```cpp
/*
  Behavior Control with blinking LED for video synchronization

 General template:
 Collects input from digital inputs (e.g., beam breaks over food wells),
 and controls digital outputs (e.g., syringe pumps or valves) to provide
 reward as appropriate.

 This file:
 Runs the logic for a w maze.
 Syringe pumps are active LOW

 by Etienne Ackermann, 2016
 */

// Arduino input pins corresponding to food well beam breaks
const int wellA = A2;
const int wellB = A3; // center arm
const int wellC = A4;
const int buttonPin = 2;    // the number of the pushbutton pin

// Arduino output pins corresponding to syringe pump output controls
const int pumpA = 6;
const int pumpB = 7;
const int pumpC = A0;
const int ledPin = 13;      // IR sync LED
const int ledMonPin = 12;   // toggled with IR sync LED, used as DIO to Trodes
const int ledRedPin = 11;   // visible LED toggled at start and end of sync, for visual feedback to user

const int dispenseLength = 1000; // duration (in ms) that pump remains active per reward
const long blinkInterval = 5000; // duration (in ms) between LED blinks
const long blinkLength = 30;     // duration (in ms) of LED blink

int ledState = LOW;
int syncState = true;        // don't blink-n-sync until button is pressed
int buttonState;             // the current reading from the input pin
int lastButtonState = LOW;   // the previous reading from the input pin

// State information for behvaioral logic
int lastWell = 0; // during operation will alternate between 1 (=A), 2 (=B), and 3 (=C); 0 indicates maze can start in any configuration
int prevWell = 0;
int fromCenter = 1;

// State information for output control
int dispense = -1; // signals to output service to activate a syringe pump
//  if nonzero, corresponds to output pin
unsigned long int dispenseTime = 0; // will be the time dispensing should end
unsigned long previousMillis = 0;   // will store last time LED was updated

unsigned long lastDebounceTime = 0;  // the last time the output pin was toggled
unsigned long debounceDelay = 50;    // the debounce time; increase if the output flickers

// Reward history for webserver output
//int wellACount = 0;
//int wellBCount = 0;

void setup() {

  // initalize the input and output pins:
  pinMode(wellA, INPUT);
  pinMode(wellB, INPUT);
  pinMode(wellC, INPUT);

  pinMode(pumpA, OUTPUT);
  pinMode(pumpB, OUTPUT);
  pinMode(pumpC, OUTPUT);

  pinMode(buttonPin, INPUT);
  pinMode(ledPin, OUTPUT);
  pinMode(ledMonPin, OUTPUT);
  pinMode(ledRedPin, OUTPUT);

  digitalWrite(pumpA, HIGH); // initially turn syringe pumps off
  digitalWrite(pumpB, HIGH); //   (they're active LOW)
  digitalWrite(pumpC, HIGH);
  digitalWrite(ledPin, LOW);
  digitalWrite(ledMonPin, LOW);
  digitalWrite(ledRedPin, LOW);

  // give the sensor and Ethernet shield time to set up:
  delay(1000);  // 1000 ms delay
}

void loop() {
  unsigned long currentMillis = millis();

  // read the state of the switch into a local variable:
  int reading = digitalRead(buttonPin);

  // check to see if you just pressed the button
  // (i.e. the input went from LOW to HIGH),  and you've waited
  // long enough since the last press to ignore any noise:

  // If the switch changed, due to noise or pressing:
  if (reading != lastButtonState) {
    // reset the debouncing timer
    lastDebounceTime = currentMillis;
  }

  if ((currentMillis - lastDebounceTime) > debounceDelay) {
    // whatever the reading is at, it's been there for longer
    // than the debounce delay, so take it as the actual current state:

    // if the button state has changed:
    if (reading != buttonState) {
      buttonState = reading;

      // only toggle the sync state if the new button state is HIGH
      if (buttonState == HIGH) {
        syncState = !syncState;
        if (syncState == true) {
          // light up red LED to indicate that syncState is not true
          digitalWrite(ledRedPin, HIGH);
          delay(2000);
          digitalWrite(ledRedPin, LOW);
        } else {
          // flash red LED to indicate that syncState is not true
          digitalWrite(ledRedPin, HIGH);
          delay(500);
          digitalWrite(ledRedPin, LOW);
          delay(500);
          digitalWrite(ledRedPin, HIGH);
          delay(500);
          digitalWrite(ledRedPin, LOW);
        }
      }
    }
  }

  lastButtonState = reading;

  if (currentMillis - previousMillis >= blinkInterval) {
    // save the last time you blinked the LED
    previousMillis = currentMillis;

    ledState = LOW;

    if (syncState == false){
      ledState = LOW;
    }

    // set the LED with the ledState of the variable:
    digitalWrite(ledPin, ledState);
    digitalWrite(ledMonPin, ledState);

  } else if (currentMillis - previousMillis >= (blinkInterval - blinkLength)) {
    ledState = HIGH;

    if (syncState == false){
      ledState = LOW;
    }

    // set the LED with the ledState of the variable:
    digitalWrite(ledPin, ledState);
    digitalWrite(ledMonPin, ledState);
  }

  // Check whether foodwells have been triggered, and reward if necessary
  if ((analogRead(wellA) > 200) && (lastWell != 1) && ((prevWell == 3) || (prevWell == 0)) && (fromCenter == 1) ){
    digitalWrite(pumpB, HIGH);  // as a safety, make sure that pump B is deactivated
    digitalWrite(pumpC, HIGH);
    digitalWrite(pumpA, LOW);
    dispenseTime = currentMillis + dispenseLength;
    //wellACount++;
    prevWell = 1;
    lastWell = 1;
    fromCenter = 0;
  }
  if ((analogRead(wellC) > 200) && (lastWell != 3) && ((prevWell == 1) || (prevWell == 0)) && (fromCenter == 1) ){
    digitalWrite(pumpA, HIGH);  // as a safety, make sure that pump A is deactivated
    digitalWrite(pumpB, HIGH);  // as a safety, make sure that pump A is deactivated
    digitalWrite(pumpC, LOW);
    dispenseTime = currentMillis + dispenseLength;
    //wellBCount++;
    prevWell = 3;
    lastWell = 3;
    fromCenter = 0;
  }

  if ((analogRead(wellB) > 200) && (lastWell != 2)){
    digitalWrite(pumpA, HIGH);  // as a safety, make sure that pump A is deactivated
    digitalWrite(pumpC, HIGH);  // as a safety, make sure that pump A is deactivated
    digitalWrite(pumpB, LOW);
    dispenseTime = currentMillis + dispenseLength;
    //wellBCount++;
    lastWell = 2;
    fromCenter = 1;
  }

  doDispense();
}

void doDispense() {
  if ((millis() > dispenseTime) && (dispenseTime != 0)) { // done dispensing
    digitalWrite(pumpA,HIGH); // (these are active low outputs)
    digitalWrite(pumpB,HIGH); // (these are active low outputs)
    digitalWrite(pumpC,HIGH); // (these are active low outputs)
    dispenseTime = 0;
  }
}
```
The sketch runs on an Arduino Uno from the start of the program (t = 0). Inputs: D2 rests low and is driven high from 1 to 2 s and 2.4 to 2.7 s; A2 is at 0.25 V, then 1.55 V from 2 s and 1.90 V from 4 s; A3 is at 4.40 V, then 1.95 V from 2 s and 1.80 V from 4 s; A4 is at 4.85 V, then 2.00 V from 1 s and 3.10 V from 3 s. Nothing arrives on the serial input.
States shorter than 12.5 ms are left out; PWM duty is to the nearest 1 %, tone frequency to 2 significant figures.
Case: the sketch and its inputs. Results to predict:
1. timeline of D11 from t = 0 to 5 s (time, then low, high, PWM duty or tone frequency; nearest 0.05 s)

0 s low; 1.05 s high; 1.55 s low; 2.05 s high; 2.55 s low
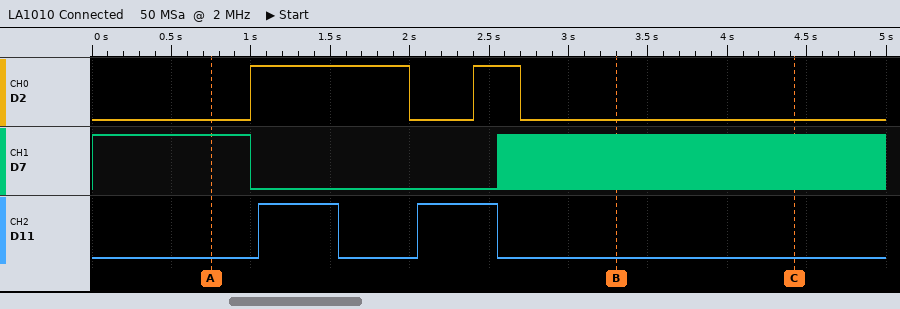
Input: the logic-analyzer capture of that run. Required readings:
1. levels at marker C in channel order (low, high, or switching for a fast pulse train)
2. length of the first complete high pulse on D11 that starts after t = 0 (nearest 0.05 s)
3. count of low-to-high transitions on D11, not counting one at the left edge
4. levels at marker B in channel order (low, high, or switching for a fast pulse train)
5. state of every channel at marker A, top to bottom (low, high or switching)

D2 low, D7 switching, D11 low
0.50 s
2
D2 low, D7 switching, D11 low
D2 low, D7 high, D11 low
